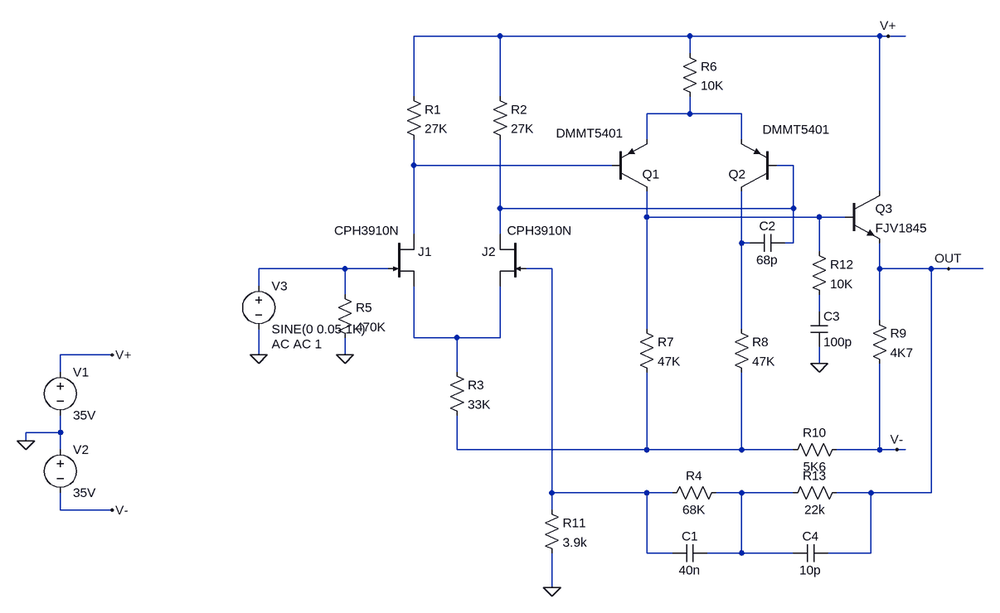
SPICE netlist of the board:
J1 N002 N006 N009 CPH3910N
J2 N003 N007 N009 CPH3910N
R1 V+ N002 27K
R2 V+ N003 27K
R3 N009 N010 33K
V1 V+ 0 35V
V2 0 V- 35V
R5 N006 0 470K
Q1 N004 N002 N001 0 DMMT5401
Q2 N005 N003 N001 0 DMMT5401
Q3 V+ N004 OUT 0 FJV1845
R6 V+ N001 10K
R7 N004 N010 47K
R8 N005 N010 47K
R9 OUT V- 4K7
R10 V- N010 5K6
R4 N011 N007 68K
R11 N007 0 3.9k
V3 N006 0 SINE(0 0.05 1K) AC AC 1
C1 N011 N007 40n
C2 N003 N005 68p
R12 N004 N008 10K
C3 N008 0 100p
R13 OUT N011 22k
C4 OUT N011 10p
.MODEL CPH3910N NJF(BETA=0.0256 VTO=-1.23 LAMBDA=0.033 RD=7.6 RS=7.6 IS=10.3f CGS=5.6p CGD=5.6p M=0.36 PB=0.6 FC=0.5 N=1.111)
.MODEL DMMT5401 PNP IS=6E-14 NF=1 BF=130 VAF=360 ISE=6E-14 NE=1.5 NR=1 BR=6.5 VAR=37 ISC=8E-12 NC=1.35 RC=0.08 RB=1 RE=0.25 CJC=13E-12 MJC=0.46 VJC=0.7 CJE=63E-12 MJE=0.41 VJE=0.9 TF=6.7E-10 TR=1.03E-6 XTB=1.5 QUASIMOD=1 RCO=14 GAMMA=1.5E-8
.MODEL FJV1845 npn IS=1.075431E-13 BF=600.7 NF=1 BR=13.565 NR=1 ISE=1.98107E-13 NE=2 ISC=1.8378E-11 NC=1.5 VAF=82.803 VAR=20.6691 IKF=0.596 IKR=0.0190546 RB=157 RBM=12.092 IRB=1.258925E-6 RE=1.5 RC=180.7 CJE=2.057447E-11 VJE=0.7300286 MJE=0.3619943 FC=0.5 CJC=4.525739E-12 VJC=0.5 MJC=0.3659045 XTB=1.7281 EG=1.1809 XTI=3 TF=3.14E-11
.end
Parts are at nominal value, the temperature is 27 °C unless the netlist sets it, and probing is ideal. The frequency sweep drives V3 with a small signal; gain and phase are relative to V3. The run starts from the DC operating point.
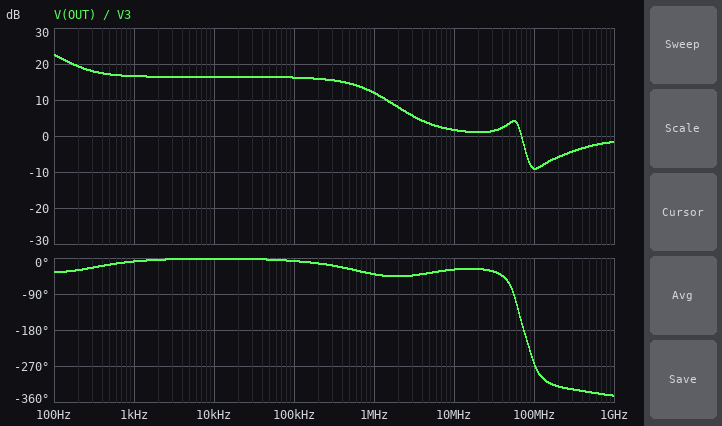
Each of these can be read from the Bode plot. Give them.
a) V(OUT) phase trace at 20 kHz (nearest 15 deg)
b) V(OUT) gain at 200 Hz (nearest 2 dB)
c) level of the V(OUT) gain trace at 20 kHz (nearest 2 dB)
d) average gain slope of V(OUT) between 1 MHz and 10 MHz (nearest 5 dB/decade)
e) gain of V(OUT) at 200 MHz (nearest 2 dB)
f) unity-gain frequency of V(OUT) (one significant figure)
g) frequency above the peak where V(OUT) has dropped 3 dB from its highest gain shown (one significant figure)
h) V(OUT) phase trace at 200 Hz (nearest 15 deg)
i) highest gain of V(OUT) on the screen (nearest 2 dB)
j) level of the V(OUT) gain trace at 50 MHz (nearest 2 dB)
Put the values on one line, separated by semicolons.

0 deg; 20 dB; 16 dB; -10 dB/decade; -6 dB; 70 MHz; 200 Hz; -30 deg; 22 dB; 4 dB
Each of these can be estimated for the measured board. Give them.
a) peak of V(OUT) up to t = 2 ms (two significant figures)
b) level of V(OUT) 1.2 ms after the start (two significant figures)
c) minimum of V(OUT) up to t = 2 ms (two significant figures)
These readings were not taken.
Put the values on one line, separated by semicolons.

380 mV; 330 mV; -320 mV
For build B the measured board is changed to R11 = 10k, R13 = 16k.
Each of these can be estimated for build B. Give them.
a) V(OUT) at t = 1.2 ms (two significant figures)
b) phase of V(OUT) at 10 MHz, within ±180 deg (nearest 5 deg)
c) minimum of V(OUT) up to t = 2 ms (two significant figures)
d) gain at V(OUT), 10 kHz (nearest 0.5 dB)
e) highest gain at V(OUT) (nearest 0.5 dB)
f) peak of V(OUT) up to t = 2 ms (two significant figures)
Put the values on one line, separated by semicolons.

130 mV; -15 deg; -120 mV; 8.5 dB; 19.5 dB; 150 mV
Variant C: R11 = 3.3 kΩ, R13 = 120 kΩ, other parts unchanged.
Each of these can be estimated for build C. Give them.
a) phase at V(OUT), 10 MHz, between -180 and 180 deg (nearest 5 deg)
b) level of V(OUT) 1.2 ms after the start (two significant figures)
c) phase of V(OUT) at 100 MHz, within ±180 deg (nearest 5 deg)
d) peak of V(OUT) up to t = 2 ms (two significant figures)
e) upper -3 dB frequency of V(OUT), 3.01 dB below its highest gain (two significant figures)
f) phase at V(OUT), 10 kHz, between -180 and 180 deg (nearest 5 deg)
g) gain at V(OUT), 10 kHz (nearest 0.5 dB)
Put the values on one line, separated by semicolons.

-35 deg; 1.8 V; 100 deg; 1.9 V; 140 Hz; -5 deg; 31.5 dB
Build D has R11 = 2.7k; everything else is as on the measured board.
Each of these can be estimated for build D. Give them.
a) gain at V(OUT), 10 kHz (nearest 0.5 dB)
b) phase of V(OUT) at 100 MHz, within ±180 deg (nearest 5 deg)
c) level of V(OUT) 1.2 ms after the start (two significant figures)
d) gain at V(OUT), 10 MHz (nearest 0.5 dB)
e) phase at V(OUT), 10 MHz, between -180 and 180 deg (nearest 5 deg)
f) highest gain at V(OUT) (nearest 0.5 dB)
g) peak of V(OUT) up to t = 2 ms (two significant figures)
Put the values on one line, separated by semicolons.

19.0 dB; 100 deg; 460 mV; 2.0 dB; -35 deg; 30.5 dB; 530 mV
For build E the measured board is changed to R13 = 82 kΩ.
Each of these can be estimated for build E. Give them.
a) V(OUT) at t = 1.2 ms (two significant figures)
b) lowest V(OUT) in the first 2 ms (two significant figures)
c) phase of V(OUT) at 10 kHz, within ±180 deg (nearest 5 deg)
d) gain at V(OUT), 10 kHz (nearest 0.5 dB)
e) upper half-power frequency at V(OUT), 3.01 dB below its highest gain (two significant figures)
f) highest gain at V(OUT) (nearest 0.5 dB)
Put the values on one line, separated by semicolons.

1.1 V; -1.1 V; -5 deg; 27.0 dB; 96 Hz; 32.0 dB
